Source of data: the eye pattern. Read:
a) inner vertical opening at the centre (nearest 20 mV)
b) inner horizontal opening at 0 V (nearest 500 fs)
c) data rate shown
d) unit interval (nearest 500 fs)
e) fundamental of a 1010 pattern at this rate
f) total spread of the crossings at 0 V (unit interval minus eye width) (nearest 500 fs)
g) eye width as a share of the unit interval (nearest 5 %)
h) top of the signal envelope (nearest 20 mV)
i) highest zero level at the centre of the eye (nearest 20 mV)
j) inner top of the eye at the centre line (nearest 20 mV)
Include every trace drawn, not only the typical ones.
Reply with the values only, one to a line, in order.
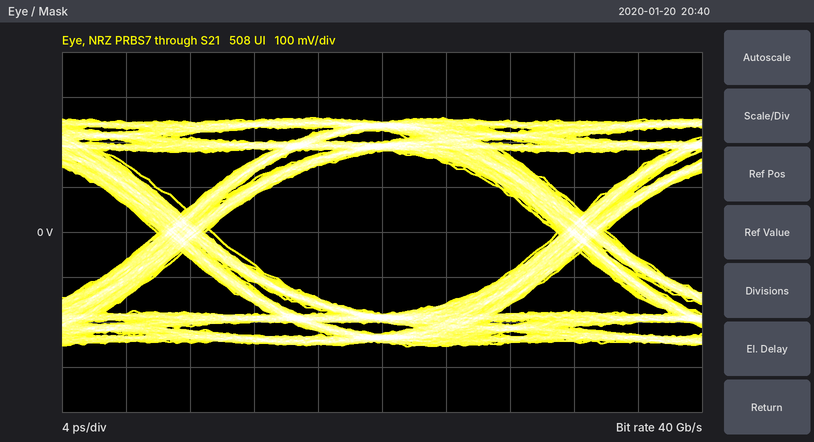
360 mV
21.5 ps
40 Gb/s
25.0 ps
20 GHz
3.5 ps
85 %
260 mV
-180 mV
180 mV
